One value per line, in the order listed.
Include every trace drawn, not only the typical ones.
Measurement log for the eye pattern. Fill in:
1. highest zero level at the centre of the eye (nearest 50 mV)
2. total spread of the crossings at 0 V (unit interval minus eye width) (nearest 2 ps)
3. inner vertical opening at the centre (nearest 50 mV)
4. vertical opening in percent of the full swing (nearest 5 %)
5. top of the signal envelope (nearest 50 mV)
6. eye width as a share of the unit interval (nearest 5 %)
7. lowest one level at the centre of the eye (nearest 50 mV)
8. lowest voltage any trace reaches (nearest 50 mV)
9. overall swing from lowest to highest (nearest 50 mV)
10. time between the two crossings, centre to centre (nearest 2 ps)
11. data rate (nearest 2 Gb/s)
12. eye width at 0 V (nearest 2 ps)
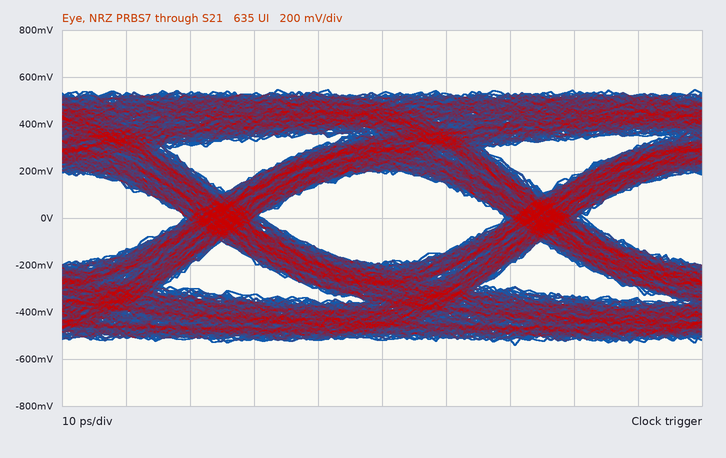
-200 mV
12 ps
400 mV
35 %
550 mV
75 %
200 mV
-550 mV
1.10 V
50 ps
20 Gb/s
38 ps
